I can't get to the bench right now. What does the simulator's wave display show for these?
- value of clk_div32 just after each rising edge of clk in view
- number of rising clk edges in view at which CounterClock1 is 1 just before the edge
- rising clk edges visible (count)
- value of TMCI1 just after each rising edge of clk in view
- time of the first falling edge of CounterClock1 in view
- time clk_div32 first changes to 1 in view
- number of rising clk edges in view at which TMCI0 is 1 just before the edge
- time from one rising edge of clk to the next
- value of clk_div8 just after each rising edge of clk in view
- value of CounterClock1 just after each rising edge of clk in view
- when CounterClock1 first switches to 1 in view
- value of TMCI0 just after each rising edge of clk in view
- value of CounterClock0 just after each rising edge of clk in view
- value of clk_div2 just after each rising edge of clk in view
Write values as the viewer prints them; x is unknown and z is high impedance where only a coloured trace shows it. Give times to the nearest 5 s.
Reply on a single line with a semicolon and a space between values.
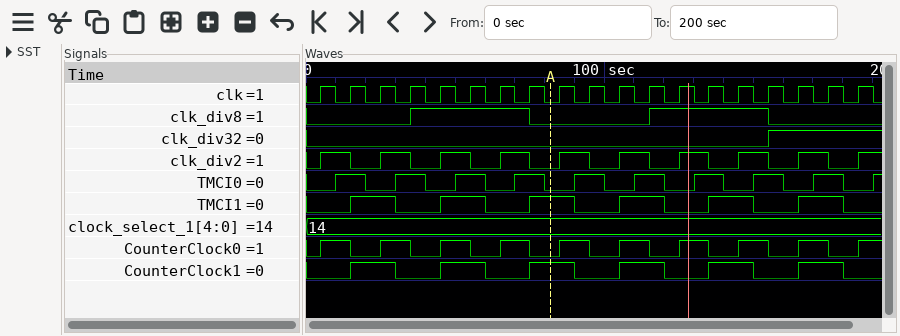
0 0 0 0 0 0 0 0 0 0 0 0 0 0 0 1 1 1 1; 6; 19; 0 1 1 0 1 1 0 1 1 0 1 1 0 1 1 0 1 1 0; 30 s; 155 s; 9; 10 s; 0 0 0 1 1 1 1 0 0 0 0 1 1 1 1 0 0 0 0; 0 1 1 0 1 1 0 1 1 0 1 1 0 1 1 0 1 1 0; 15 s; 0 1 0 1 0 1 0 1 0 1 0 1 0 1 0 1 0 1 0; 1 0 1 0 1 0 1 0 1 0 1 0 1 0 1 0 1 0 1; 1 0 1 0 1 0 1 0 1 0 1 0 1 0 1 0 1 0 1
